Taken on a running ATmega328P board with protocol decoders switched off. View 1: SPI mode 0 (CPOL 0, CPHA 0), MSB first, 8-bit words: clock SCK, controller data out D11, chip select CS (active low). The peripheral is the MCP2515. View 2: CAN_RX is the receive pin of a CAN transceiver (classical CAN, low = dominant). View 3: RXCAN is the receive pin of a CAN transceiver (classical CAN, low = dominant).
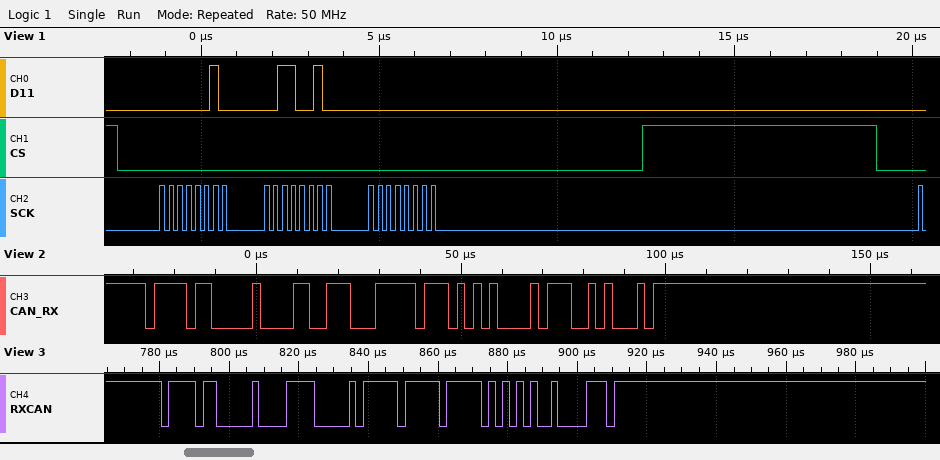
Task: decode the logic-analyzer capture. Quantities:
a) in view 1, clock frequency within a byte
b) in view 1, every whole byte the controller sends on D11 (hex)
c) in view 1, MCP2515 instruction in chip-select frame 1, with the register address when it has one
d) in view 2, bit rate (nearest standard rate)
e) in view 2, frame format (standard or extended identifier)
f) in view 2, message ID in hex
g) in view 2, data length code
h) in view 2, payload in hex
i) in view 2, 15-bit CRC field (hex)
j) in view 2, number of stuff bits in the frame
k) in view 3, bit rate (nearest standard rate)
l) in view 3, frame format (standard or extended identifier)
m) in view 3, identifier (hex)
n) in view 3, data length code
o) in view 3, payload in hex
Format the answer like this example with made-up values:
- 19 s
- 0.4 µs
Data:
- 4 MHz
- 02 32 00
- WRITE 0x32
- 500 kbit/s
- standard
- 0x7B0
- 3
- 38 FF 54
- 0x1728
- 2
- 500 kbit/s
- standard
- 0x7B0
- 3
- C0 FF FF
